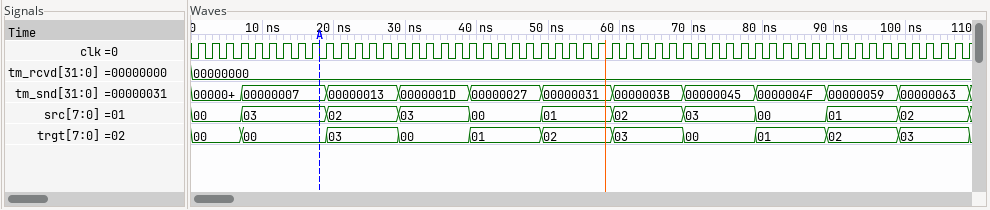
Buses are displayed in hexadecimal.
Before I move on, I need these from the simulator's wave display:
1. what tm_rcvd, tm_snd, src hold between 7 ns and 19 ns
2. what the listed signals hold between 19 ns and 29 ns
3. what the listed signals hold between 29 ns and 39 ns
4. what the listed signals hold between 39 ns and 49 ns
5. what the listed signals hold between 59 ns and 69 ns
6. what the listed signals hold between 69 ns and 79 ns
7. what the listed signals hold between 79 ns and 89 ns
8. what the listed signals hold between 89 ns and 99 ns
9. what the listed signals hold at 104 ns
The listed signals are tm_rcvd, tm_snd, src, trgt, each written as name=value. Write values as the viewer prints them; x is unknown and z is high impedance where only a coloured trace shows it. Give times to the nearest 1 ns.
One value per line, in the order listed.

tm_rcvd=00000000, tm_snd=00000007, src=03
tm_rcvd=00000000, tm_snd=00000013, src=02, trgt=03
tm_rcvd=00000000, tm_snd=0000001D, src=03, trgt=00
tm_rcvd=00000000, tm_snd=00000027, src=00, trgt=01
tm_rcvd=00000000, tm_snd=0000003B, src=02, trgt=03
tm_rcvd=00000000, tm_snd=00000045, src=03, trgt=00
tm_rcvd=00000000, tm_snd=0000004F, src=00, trgt=01
tm_rcvd=00000000, tm_snd=00000059, src=01, trgt=02
tm_rcvd=00000000, tm_snd=00000063, src=02, trgt=03
